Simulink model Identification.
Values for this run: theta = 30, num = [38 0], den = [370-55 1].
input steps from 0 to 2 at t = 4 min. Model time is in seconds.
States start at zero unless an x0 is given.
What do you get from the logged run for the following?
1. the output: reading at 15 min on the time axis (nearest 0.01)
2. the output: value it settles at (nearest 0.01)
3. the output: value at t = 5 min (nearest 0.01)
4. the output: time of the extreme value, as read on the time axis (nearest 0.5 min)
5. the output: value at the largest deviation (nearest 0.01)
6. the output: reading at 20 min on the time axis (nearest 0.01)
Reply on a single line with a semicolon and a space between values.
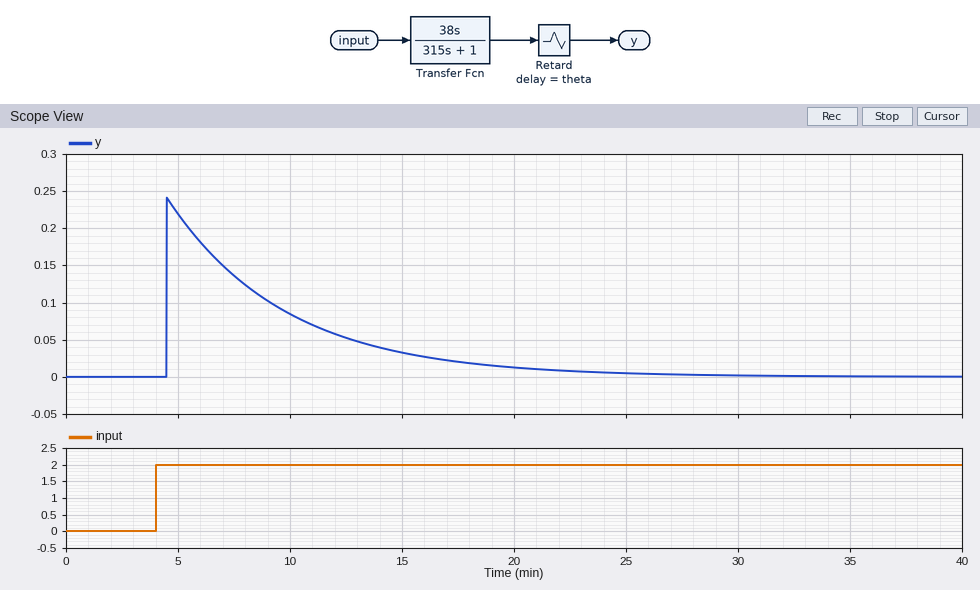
0.03; 0.00; 0.22; 4.5 min; 0.24; 0.01
